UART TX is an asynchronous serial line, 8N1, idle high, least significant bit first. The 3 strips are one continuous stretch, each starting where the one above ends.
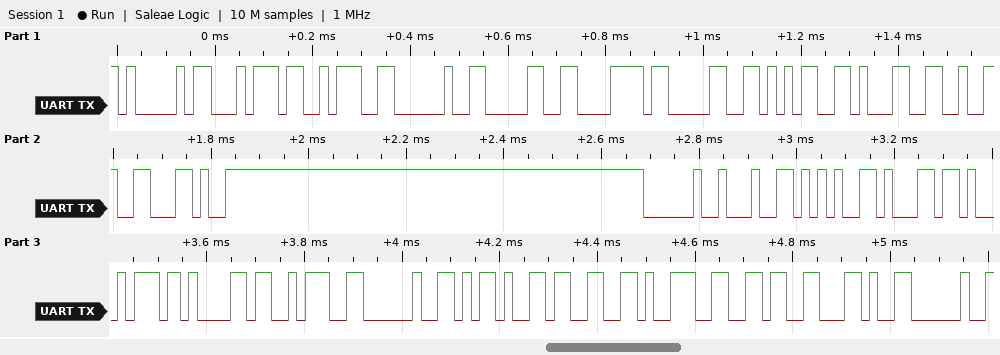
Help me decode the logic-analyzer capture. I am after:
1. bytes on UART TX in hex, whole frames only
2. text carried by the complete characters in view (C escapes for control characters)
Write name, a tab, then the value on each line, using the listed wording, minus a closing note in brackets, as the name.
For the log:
bytes on UART TX in hex, whole frames only	41 74 3A 20 30 78 30 35 31 32 2C 20 64 65 6C 74 61 3A 20 2D 33 39 36 2C 20
text carried by the complete characters in view	"At: 0x0512, delta: -396, "
